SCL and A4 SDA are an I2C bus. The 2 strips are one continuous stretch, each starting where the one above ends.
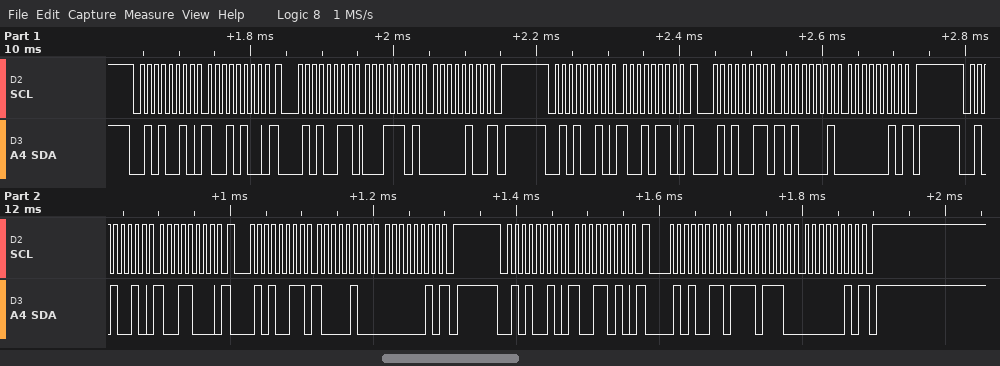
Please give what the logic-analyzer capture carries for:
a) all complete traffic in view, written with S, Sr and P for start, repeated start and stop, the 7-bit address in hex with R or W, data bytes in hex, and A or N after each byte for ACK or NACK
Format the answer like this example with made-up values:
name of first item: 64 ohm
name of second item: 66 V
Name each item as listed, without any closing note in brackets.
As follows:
all complete traffic in view, written with S, Sr and P for start, repeated start and stop, the 7-bit address in hex with R or W, data bytes in hex, and A or N after each byte for ACK or NACK: S 29W A 94 A Sr 29R A 1D A 04 N P S 29W A 96 A Sr 29R A A1 A 02 N P S 29W A 98 A Sr 29R A 84 A 02 N P S 29W A 9A A Sr 29R A EE A 02 N P
